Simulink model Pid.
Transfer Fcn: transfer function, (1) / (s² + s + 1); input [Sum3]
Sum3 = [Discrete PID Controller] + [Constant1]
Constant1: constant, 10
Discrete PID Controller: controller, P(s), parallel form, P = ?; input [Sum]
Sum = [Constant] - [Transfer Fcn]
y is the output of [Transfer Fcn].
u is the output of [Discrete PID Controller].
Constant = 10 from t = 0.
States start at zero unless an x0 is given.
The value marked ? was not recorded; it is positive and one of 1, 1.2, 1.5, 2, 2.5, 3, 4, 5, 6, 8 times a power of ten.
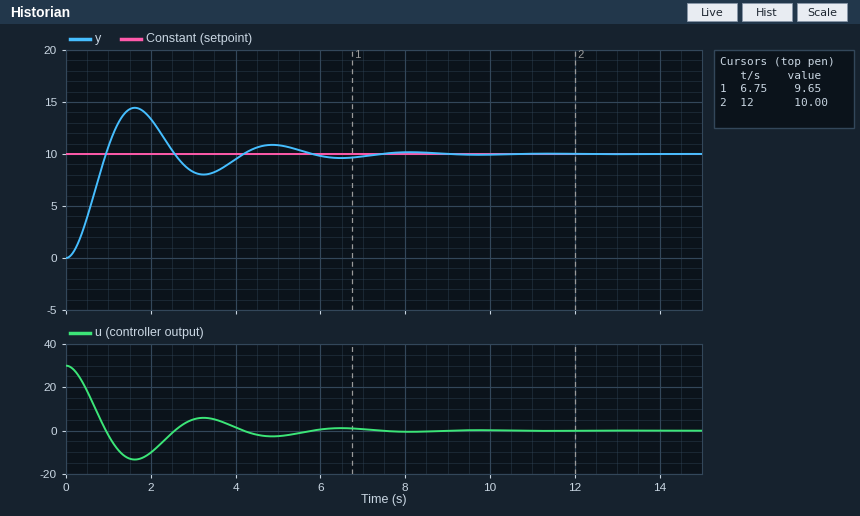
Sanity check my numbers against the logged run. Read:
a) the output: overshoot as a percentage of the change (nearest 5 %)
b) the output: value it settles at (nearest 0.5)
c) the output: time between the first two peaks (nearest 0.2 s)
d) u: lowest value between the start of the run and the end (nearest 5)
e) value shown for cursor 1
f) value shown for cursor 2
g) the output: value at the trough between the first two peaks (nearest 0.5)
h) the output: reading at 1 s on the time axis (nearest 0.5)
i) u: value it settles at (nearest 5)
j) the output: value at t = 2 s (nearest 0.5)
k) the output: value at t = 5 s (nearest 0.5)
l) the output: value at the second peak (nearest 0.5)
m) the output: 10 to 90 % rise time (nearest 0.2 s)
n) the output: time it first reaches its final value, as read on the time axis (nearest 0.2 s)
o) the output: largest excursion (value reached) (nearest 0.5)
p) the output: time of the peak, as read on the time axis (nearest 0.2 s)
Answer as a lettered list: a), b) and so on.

a) 45 %
b) 10.0
c) 3.2 s
d) -15
e) 9.65
f) 10.00
g) 8.0
h) 10.5
i) 0
j) 13.5
k) 11.0
l) 11.0
m) 0.6 s
n) 1.0 s
o) 14.5
p) 1.6 s
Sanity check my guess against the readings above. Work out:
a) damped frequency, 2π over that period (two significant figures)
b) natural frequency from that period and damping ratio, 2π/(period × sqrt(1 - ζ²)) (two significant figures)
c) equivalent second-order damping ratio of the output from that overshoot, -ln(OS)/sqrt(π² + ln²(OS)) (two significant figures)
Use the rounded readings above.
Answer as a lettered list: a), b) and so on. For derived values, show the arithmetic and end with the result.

a) 2π / 3.2 = 2.0 rad/s
b) 2π / (3.2 × sqrt(1 - 0.25²)) = 2.0 rad/s
c) ln(0.45) = -0.799; 0.799 / sqrt(9.870 + 0.638) = 0.25
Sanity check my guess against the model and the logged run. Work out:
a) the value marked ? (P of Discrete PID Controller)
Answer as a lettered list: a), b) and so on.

a) 3
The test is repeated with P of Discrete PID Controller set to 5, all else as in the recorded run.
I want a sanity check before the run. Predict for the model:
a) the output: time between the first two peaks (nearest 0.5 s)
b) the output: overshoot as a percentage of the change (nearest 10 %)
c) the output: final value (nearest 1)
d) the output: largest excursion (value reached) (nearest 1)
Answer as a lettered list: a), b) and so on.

a) 2.5 s
b) 50 %
c) 10
d) 15
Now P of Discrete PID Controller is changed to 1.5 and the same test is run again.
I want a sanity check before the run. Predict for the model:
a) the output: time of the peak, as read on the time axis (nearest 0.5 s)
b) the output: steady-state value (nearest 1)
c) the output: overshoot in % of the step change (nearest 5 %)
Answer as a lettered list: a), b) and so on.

a) 2.0 s
b) 10
c) 35 %
